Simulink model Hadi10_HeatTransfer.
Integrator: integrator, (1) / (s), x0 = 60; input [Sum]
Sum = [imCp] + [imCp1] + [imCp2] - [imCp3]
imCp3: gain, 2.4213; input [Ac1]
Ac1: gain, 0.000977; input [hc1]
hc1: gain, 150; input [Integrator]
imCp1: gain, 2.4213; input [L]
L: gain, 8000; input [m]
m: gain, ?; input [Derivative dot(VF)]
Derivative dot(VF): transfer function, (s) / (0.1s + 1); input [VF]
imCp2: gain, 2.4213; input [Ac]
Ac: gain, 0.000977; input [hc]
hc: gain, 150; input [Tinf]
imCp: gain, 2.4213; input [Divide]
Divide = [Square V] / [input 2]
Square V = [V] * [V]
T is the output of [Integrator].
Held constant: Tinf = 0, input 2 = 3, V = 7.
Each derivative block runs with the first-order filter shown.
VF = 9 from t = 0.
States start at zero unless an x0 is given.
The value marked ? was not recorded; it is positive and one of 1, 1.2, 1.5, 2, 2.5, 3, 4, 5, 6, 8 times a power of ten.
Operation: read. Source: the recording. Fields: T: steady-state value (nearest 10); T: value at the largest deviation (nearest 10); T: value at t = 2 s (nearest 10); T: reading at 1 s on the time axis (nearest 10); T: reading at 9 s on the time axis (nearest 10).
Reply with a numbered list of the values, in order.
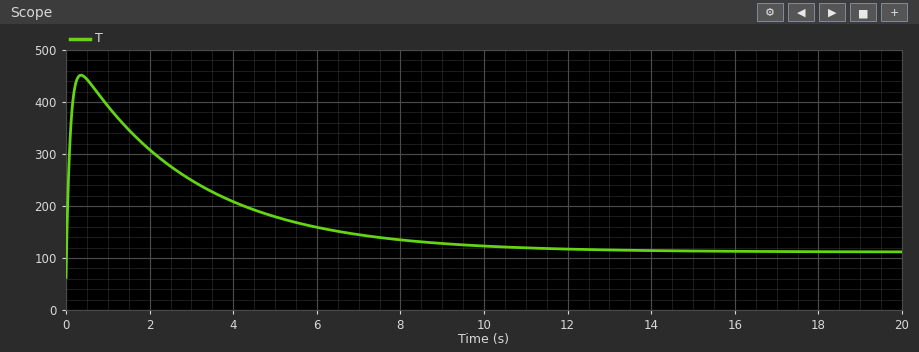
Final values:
1. 110
2. 450
3. 310
4. 390
5. 130
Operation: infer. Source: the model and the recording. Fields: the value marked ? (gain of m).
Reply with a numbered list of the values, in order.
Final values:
1. 0.0025
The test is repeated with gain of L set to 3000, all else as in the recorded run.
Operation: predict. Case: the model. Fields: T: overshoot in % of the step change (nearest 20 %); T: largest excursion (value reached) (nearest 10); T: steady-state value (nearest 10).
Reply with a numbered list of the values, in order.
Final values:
1. 200 %
2. 210
3. 110
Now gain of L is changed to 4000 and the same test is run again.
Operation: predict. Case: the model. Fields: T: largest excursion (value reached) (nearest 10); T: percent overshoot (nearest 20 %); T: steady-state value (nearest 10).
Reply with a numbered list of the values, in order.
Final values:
1. 260
2. 280 %
3. 110
